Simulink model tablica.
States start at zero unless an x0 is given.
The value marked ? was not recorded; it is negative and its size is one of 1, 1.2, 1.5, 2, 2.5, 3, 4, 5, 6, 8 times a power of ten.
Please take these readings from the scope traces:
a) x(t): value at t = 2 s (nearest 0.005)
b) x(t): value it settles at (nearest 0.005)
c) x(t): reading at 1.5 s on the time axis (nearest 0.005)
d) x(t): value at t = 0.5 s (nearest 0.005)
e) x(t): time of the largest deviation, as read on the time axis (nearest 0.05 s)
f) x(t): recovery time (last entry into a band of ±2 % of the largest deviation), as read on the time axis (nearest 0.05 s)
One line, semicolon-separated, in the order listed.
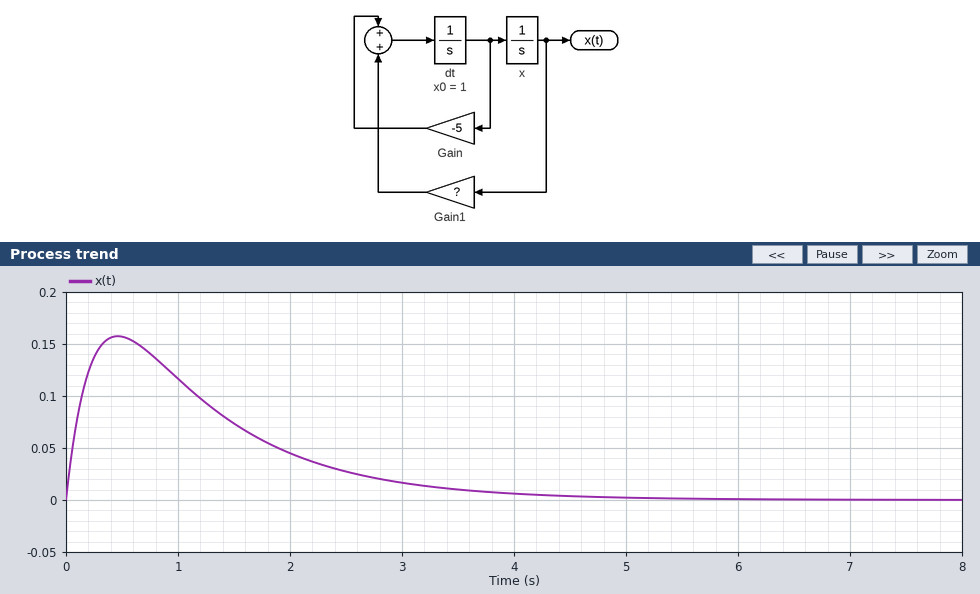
0.045; 0.000; 0.075; 0.155; 0.45 s; 4.65 s
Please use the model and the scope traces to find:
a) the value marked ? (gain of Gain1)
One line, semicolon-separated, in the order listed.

-4
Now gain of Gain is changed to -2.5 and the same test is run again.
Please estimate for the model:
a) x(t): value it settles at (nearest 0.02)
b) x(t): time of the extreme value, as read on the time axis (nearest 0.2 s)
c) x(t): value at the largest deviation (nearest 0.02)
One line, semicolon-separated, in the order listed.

0.00; 0.6 s; 0.24
